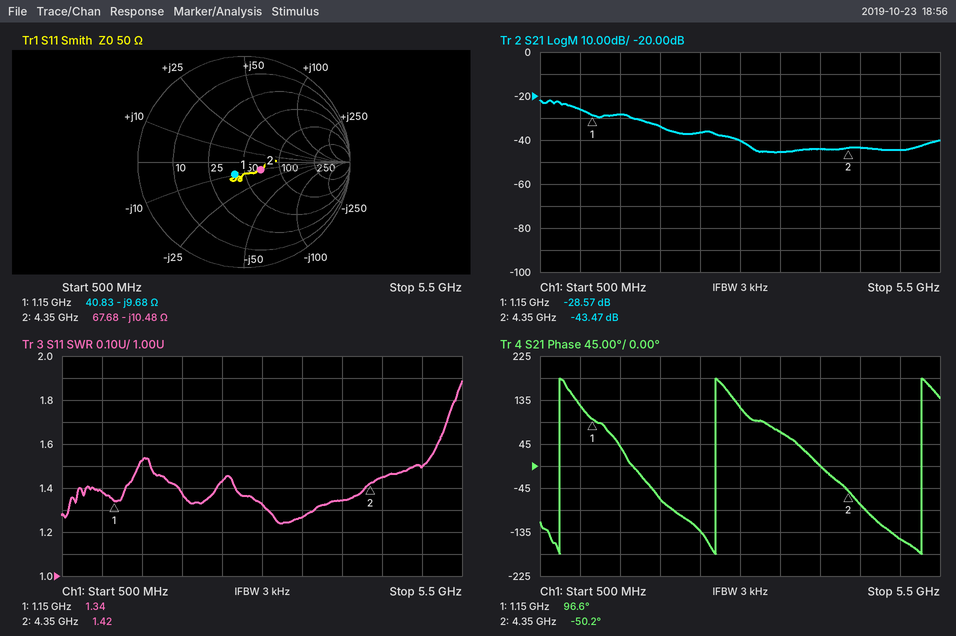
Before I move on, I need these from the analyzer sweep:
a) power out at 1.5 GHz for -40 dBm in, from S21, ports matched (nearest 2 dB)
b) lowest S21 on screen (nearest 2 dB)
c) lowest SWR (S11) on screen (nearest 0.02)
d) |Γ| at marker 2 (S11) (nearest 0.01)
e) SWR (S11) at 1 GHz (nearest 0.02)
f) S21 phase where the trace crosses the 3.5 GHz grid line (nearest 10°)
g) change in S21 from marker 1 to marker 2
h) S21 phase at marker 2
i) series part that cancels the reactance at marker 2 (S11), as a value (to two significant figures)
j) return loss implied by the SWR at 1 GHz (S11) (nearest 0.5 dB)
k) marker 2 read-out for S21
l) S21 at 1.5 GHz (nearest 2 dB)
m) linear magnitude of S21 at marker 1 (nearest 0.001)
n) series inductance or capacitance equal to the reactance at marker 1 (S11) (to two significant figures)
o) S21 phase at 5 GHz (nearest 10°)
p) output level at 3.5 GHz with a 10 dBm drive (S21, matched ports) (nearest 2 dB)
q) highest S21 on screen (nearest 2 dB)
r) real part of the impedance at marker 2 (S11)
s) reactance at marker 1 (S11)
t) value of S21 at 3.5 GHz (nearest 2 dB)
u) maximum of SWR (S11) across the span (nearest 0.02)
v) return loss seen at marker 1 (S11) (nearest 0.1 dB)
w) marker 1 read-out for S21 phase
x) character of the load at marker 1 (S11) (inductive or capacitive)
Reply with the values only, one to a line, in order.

-68 dBm
-46 dB
1.24
0.17
1.38
70°
-14.90 dB
-50.2°
380 pH
16.0 dB
-43.47 dB
-28 dB
0.037
14 pF
-150°
-36 dBm
-22 dB
67.68 Ω
-9.68 Ω
-46 dB
1.88
16.7 dB
96.6°
capacitive
